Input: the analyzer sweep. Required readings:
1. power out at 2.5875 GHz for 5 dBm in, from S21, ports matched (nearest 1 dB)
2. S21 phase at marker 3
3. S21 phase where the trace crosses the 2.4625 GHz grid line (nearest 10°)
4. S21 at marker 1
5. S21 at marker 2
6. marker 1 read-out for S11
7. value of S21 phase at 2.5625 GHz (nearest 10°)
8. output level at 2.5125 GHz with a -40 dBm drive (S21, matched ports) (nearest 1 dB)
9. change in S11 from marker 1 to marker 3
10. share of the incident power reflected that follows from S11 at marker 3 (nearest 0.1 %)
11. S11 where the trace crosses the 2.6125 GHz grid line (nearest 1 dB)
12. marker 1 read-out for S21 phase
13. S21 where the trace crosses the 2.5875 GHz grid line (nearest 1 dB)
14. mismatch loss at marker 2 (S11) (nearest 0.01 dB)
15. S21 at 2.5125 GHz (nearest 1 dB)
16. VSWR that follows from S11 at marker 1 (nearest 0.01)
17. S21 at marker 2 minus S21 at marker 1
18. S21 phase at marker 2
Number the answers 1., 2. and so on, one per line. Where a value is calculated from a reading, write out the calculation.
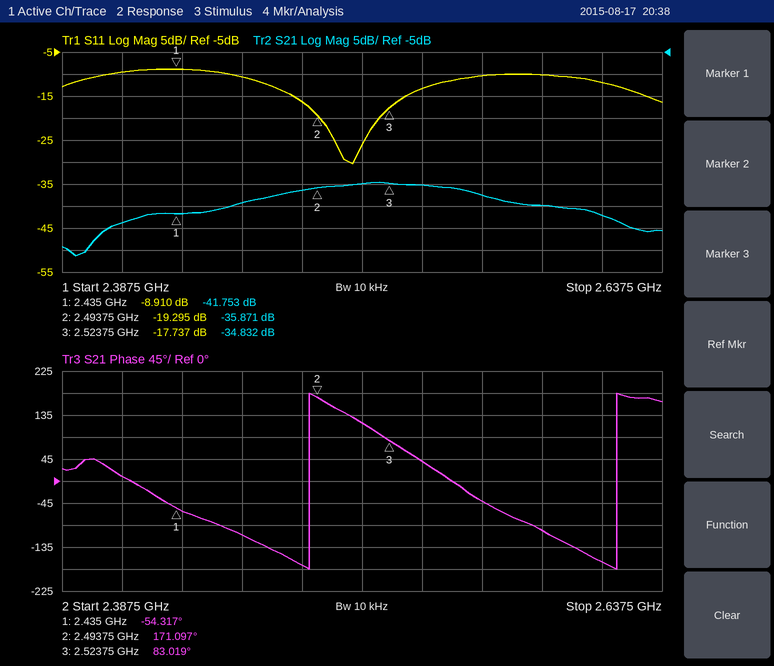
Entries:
1. 5 dBm + (-40 dB) = -35 dBm
2. 83.019°
3. -110°
4. -41.753 dB
5. -35.871 dB
6. -8.910 dB
7. -40°
8. -40 dBm + (-35 dB) = -75 dBm
9. -17.737 − (-8.91) = -8.827 dB
10. 10^(-17.737/10) ≈ 1.7 %
11. -12 dB
12. -54.317°
13. -40 dB
14. −10 log10(1 − 10^(-19.295/10)) ≈ 0.05 dB
15. -35 dB
16. (1 + 0.3585)/(1 − 0.3585) ≈ 2.12
17. -35.871 − (-41.753) = 5.882 dB
18. 171.097°
